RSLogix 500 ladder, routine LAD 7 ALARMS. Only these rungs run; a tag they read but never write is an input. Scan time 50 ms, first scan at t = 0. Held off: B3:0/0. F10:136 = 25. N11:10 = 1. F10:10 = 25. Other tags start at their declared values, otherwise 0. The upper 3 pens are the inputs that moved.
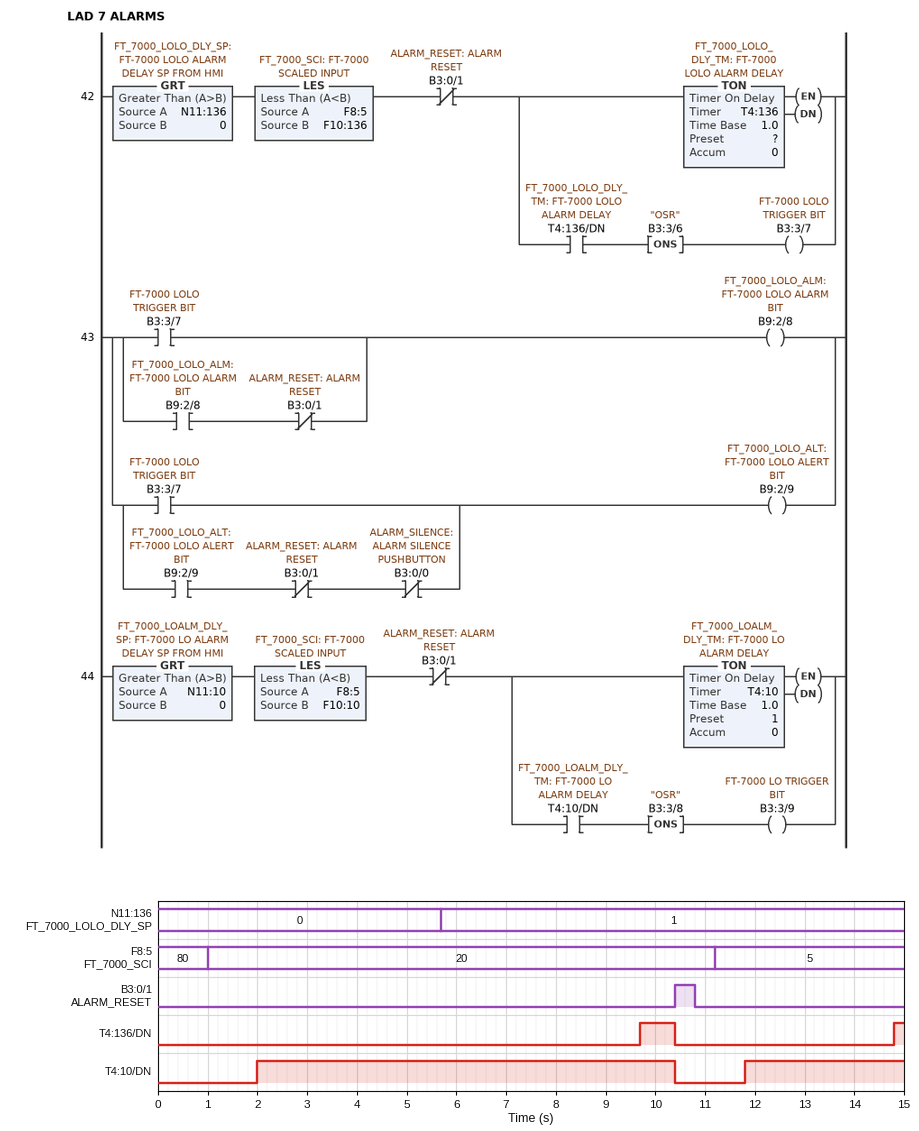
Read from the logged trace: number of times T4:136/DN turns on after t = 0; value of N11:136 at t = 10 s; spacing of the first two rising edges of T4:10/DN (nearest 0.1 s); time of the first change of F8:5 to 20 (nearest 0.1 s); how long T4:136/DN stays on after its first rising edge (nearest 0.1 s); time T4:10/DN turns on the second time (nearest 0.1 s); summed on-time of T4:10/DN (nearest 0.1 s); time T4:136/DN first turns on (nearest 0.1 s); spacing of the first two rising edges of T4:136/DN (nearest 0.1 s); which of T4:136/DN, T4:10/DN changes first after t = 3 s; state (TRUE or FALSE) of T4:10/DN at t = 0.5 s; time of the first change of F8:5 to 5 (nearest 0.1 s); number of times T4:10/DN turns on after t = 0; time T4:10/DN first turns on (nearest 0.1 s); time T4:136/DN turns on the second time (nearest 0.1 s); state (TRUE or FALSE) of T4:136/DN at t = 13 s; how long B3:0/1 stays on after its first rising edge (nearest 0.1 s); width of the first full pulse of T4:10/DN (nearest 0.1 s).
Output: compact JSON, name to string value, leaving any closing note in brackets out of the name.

{"number of times T4:136/DN turns on after t = 0": "2", "value of N11:136 at t = 10 s": "1", "spacing of the first two rising edges of T4:10/DN": "9.8 s", "time of the first change of F8:5 to 20": "1.0 s", "how long T4:136/DN stays on after its first rising edge": "0.7 s", "time T4:10/DN turns on the second time": "11.8 s", "summed on-time of T4:10/DN": "11.6 s", "time T4:136/DN first turns on": "9.7 s", "spacing of the first two rising edges of T4:136/DN": "5.1 s", "which of T4:136/DN, T4:10/DN changes first after t = 3 s": "T4:136/DN", "state (TRUE or FALSE) of T4:10/DN at t = 0.5 s": "FALSE", "time of the first change of F8:5 to 5": "11.2 s", "number of times T4:10/DN turns on after t = 0": "2", "time T4:10/DN first turns on": "2.0 s", "time T4:136/DN turns on the second time": "14.8 s", "state (TRUE or FALSE) of T4:136/DN at t = 13 s": "FALSE", "how long B3:0/1 stays on after its first rising edge": "0.4 s", "width of the first full pulse of T4:10/DN": "8.4 s"}
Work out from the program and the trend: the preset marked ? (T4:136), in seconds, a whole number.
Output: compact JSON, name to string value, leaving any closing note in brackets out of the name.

{"the preset marked ? (T4:136), in seconds, a whole number": "4 s"}
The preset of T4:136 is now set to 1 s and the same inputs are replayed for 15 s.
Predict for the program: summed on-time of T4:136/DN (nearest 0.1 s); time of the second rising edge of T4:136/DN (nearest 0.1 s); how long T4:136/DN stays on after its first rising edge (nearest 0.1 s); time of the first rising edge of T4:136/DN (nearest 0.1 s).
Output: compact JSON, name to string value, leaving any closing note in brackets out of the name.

{"summed on-time of T4:136/DN": "6.9 s", "time of the second rising edge of T4:136/DN": "11.8 s", "how long T4:136/DN stays on after its first rising edge": "3.7 s", "time of the first rising edge of T4:136/DN": "6.7 s"}
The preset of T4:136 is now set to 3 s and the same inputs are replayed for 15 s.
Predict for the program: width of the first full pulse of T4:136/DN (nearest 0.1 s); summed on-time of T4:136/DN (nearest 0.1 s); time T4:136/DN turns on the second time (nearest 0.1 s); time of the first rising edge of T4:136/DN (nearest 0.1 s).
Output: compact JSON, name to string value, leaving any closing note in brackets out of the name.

{"width of the first full pulse of T4:136/DN": "1.7 s", "summed on-time of T4:136/DN": "2.9 s", "time T4:136/DN turns on the second time": "13.8 s", "time of the first rising edge of T4:136/DN": "8.7 s"}
